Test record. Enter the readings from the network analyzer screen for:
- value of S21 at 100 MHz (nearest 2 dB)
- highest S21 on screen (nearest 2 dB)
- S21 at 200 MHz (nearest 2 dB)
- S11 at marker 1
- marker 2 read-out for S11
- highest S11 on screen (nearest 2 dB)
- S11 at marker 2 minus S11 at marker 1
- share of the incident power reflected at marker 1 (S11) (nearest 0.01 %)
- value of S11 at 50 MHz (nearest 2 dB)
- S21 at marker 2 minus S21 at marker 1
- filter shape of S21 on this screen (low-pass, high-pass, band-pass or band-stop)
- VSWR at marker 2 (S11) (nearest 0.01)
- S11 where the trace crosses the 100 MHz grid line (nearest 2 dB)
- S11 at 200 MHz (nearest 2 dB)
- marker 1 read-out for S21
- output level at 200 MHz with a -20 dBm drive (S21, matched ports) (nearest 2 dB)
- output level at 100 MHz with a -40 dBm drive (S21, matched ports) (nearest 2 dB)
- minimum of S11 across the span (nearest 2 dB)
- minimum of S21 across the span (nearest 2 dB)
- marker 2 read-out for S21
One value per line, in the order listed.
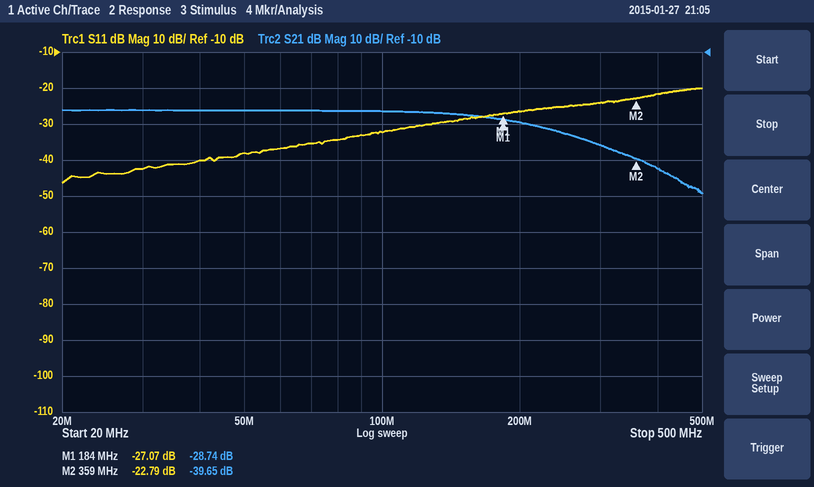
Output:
-26 dB
-26 dB
-30 dB
-27.07 dB
-22.79 dB
-20 dB
4.28 dB
0.20 %
-38 dB
-10.91 dB
low-pass
1.16
-32 dB
-26 dB
-28.74 dB
-50 dBm
-66 dBm
-46 dB
-50 dB
-39.65 dB
